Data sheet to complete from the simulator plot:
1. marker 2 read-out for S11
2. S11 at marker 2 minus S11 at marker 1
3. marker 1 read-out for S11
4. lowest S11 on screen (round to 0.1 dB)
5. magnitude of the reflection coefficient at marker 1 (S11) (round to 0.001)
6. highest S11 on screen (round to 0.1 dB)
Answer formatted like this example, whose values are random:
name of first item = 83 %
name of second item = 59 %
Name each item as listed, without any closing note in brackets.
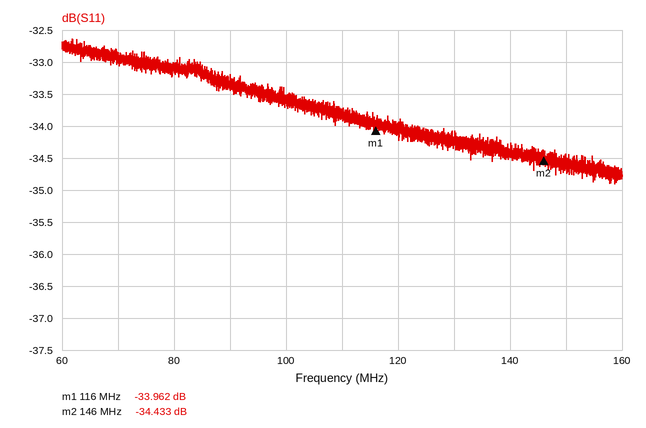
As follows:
marker 2 read-out for S11 = -34.433 dB
S11 at marker 2 minus S11 at marker 1 = -0.471 dB
marker 1 read-out for S11 = -33.962 dB
lowest S11 on screen = -34.9 dB
magnitude of the reflection coefficient at marker 1 (S11) = 0.020
highest S11 on screen = -32.6 dB
